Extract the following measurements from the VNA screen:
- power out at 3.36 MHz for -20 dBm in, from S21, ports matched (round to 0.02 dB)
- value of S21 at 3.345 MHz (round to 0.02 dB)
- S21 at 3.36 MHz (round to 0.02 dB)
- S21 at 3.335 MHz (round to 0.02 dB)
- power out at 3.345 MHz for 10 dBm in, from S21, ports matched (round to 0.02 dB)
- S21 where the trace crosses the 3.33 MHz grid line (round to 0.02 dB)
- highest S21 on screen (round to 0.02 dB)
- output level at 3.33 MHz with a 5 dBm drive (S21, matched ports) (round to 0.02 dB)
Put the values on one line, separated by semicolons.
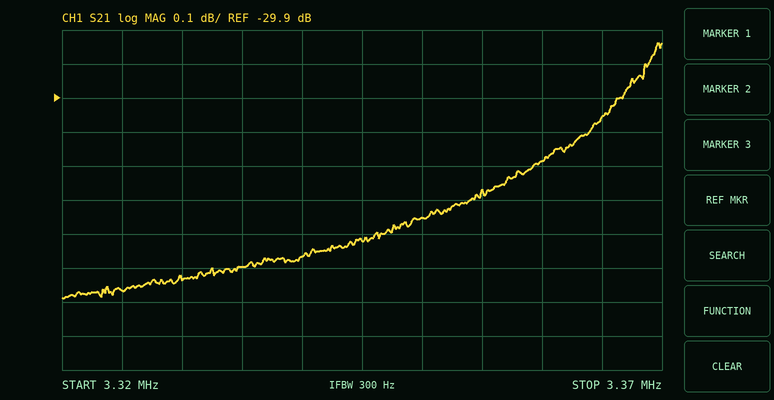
-50.08 dBm; -30.32 dB; -30.08 dB; -30.40 dB; -20.32 dBm; -30.44 dB; -29.74 dB; -25.44 dBm
